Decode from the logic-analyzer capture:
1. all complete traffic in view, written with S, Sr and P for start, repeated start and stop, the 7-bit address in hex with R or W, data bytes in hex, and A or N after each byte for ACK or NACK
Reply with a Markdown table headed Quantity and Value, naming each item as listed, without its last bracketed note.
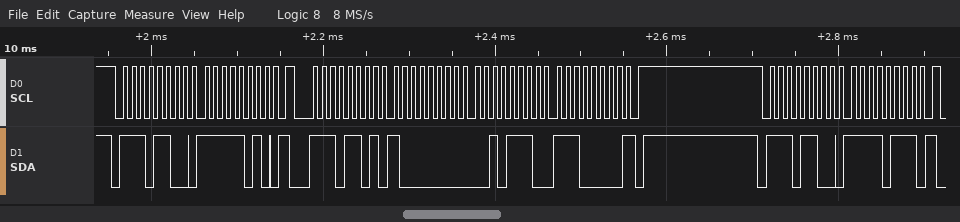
| Quantity | Value |
|---|---|
| all complete traffic in view, written with S, Sr and P for start, repeated start and stop, the 7-bit address in hex with R or W, data bytes in hex, and A or N after each byte for ACK or NACK | S 76W A FA A Sr 76R A 80 A 2E A E0 N P S 76W A F7 A |
